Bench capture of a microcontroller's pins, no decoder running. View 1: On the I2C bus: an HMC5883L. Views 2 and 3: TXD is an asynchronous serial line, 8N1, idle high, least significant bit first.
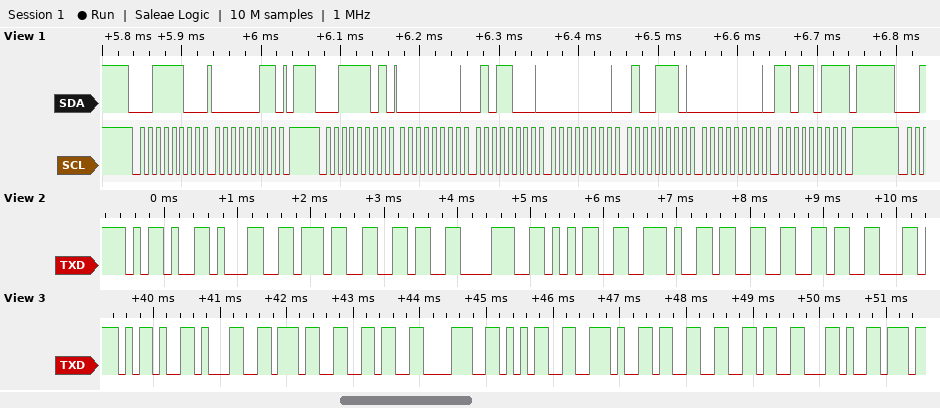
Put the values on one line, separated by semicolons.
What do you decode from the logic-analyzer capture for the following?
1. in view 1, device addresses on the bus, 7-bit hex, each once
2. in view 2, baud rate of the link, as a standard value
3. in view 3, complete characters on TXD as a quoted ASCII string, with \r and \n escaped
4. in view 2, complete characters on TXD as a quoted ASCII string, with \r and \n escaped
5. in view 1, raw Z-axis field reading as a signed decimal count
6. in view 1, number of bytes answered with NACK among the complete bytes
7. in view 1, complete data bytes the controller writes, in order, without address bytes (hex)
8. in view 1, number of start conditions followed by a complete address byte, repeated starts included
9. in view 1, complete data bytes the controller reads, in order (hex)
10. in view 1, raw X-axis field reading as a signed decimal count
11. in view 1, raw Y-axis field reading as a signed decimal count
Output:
0x1E; 9600 baud; "-17685.36,"; "-17685.36"; 78; 1; 03; 2; 00 58 00 4E 00 DB; 88; 219
